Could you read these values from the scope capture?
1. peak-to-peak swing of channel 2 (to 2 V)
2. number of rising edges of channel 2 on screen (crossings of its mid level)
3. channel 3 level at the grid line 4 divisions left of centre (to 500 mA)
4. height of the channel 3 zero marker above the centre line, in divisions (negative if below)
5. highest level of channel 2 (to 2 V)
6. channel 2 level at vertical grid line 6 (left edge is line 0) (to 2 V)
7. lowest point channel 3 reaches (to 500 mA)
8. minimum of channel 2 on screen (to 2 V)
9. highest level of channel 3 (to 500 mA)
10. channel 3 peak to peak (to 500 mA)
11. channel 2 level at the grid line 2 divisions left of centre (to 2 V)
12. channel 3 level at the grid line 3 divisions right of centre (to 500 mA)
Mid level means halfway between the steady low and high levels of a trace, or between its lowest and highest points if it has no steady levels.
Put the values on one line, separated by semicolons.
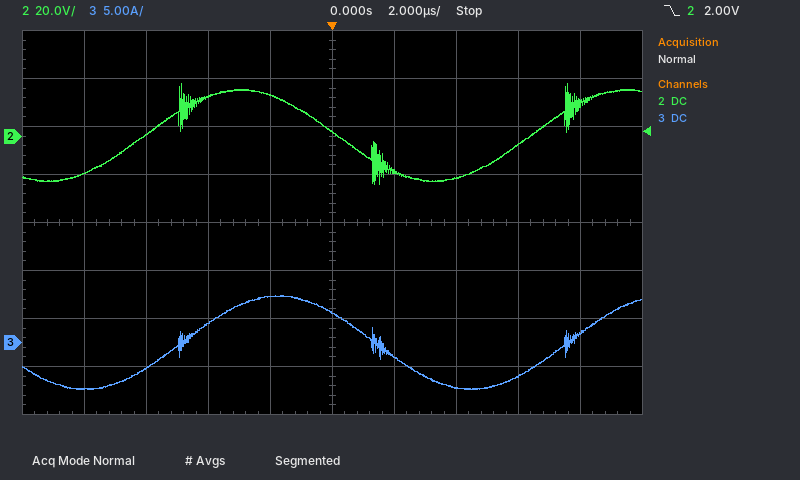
42 V; 2; -5.0 A; -2.5 div; 22 V; -14 V; -5.0 A; -20 V; 5.0 A; 10.0 A; 16 V; -3.5 A
